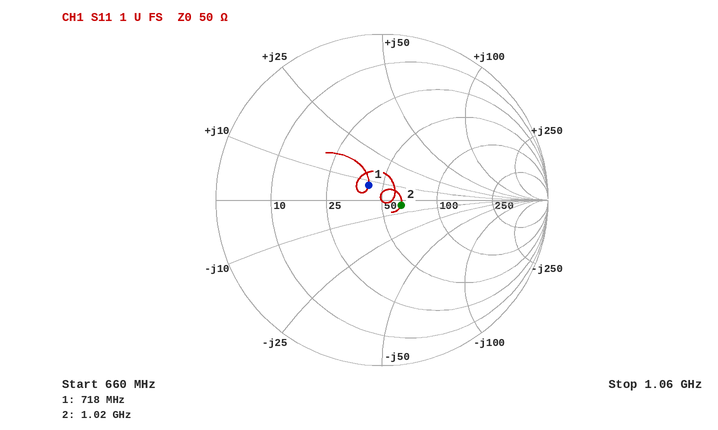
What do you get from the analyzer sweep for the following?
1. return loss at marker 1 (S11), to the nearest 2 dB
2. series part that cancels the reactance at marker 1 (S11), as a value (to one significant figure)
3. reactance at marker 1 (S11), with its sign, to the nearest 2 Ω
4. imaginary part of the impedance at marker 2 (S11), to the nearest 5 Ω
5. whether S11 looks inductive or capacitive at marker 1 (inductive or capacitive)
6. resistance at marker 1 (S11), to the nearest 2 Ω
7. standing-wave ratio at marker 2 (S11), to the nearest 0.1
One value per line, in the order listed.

18 dB
30 pF
+8 Ω
-5 Ω
inductive
42 Ω
1.3
